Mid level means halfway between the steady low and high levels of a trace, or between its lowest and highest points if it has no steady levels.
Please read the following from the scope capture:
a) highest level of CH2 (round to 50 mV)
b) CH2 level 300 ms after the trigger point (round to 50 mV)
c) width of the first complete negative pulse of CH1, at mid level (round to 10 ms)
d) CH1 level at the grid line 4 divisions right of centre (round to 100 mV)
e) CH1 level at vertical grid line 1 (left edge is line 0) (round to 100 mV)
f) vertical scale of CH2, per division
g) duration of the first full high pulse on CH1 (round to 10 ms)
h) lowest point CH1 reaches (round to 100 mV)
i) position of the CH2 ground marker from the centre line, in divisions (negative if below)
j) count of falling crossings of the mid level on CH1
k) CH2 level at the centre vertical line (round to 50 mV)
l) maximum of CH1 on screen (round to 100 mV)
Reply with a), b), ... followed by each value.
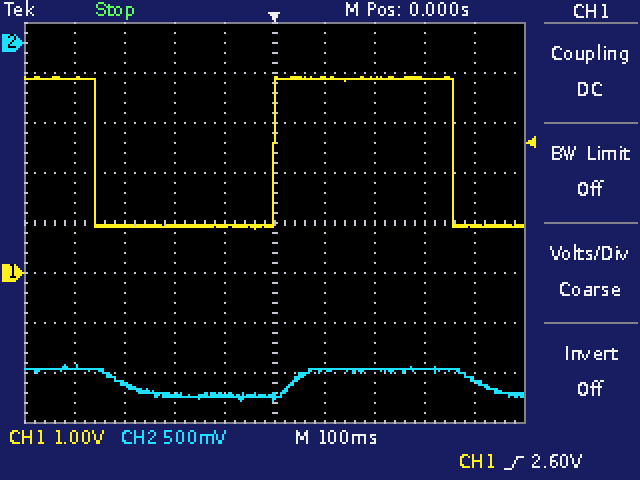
a) -3.20 V
b) -3.25 V
c) 360 ms
d) 900 mV
e) 3.9 V
f) 500 mV
g) 360 ms
h) 900 mV
i) +3.6 div
j) 2
k) -3.55 V
l) 3.9 V
